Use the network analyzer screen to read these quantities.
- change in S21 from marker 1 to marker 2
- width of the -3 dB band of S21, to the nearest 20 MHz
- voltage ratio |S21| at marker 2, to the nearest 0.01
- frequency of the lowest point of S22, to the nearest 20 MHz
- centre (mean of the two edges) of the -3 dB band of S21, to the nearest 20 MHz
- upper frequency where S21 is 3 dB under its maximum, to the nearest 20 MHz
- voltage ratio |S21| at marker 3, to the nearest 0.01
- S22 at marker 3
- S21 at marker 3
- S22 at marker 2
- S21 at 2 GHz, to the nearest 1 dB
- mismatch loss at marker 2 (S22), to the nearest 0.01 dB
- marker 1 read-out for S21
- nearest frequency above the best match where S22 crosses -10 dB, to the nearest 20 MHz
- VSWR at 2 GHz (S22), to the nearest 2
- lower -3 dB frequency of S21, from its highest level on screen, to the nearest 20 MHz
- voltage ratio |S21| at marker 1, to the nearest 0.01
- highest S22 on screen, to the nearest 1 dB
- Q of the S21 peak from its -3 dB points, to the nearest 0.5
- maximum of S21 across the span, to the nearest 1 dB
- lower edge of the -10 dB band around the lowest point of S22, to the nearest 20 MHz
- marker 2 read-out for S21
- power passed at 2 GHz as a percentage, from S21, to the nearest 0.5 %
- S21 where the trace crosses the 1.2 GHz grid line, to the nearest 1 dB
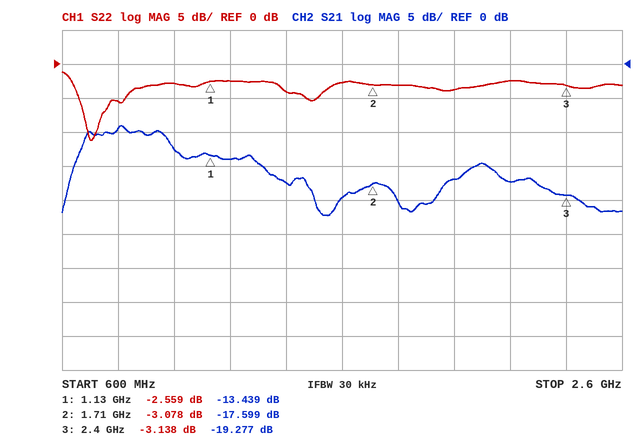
-4.160 dB
320 MHz
0.13
700 MHz
840 MHz
1.00 GHz
0.11
-3.138 dB
-19.277 dB
-3.078 dB
-17 dB
2.94 dB
-13.439 dB
720 MHz
4
680 MHz
0.21
-1 dB
2.5
-9 dB
700 MHz
-17.599 dB
2.0 %
-14 dB
